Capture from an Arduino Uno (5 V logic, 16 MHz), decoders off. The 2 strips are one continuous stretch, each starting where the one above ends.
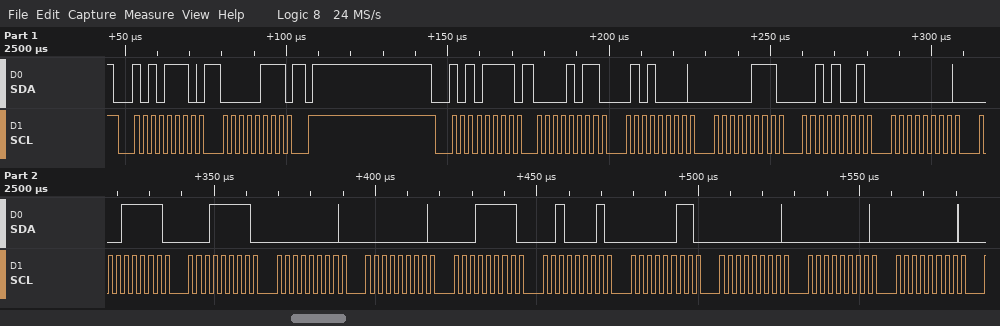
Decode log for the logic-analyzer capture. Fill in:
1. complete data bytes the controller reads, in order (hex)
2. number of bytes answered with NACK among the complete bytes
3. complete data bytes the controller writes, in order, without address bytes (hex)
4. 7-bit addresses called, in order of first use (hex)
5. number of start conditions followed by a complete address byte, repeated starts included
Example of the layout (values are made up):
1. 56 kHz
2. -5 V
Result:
1. 0B 50 07 29 00 1F 1F 00 00 1F 21 03 00 00 00
2. 0
3. 07
4. 0x57
5. 2
